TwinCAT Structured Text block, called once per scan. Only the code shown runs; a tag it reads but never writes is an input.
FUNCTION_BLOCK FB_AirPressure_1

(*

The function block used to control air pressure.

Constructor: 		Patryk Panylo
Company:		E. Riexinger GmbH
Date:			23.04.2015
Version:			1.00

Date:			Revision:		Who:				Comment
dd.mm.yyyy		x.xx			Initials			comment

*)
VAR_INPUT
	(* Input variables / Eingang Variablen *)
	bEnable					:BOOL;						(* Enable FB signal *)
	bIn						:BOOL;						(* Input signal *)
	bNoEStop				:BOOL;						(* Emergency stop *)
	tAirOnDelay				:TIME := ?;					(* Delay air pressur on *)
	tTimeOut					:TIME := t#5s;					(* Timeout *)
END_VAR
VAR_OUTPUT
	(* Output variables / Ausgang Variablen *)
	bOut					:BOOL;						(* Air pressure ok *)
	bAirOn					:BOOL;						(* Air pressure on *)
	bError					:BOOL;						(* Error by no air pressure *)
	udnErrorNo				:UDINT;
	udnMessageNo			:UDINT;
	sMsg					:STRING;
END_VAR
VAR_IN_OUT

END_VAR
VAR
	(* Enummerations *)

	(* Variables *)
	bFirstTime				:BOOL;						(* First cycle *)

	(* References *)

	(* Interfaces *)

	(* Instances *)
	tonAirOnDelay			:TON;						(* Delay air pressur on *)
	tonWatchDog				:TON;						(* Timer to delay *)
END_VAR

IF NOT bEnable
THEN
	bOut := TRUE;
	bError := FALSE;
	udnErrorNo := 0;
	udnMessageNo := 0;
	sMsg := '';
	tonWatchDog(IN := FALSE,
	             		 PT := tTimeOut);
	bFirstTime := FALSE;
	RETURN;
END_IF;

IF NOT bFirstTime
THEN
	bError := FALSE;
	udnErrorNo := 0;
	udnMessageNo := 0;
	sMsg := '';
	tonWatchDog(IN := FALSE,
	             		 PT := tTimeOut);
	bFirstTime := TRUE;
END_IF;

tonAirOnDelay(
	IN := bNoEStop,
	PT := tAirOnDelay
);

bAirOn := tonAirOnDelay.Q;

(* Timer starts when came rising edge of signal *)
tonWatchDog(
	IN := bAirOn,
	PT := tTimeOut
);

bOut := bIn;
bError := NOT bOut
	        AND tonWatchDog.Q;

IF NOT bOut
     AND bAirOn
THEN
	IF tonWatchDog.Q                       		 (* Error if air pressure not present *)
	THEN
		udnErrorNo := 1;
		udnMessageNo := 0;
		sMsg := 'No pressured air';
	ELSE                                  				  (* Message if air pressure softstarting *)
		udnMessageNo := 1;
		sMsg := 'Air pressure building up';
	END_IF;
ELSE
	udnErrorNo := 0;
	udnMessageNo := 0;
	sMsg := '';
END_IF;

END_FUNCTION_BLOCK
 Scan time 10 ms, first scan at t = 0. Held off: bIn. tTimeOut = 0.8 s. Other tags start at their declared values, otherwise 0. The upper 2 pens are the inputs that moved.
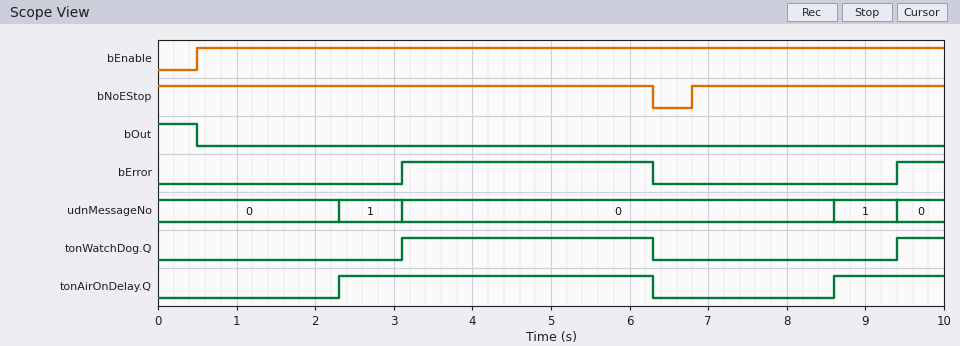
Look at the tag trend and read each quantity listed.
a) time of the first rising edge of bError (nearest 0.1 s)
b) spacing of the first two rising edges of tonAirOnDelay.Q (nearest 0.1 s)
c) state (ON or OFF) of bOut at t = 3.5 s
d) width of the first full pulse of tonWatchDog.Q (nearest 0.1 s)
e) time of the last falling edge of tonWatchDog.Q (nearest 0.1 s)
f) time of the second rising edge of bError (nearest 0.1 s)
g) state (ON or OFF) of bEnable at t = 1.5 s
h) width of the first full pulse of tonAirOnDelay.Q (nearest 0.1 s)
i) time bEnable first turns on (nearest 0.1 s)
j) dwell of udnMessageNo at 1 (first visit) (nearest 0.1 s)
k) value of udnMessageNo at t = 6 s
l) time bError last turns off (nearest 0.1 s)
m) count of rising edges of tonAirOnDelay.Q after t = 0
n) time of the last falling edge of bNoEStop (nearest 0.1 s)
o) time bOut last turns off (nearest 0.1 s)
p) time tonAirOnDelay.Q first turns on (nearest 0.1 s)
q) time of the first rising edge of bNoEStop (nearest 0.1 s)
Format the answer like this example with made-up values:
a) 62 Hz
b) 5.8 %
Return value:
a) 3.1 s
b) 6.3 s
c) OFF
d) 3.2 s
e) 6.3 s
f) 9.4 s
g) ON
h) 4.0 s
i) 0.5 s
j) 0.8 s
k) 0
l) 6.3 s
m) 2
n) 6.3 s
o) 0.5 s
p) 2.3 s
q) 6.8 s
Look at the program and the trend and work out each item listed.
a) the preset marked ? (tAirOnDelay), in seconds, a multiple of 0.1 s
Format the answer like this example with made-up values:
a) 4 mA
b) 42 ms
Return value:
a) 1.8 s
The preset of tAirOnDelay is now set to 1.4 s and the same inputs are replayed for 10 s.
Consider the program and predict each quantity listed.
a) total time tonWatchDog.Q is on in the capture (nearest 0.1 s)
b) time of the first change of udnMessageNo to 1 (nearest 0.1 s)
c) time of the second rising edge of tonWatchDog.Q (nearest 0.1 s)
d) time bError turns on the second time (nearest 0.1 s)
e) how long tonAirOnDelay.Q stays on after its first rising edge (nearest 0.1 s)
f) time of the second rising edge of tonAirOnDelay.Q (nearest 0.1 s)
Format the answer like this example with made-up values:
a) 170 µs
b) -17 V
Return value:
a) 4.6 s
b) 1.9 s
c) 9.0 s
d) 9.0 s
e) 4.4 s
f) 8.2 s
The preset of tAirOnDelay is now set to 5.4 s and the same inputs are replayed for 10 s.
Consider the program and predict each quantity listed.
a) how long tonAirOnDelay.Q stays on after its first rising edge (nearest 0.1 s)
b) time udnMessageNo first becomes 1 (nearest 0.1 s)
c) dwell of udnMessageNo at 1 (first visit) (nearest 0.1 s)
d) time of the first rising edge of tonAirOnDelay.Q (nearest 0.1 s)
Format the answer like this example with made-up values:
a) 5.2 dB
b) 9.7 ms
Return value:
a) 0.4 s
b) 5.9 s
c) 0.4 s
d) 5.9 s
